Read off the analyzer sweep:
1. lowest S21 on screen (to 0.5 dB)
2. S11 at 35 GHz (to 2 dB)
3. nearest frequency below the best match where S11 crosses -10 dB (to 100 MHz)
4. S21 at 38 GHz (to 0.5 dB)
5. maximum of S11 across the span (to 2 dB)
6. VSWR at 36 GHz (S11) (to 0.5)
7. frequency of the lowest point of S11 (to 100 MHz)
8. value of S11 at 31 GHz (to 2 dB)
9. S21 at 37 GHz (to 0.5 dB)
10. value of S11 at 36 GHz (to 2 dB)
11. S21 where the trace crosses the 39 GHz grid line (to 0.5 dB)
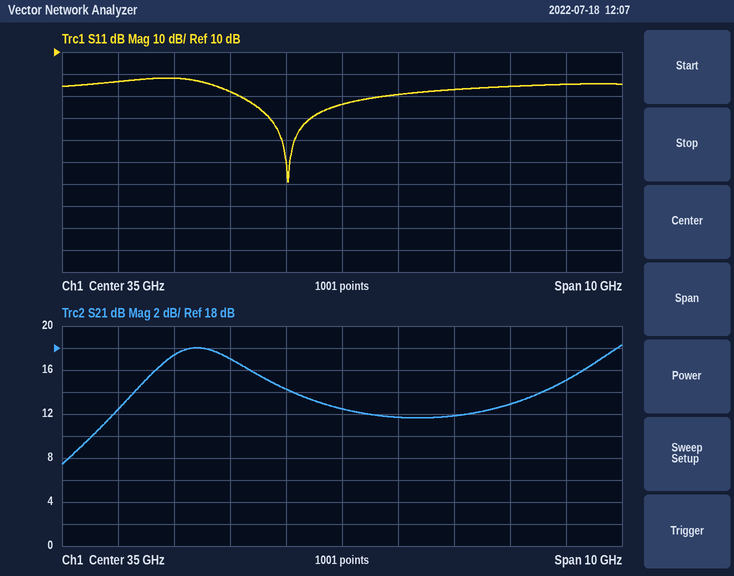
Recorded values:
7.5 dB
-14 dB
33.2 GHz
13.0 dB
-2 dB
2.0
34.0 GHz
-4 dB
12.0 dB
-10 dB
15.0 dB
